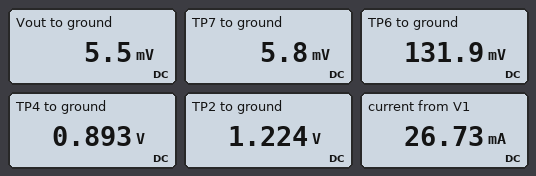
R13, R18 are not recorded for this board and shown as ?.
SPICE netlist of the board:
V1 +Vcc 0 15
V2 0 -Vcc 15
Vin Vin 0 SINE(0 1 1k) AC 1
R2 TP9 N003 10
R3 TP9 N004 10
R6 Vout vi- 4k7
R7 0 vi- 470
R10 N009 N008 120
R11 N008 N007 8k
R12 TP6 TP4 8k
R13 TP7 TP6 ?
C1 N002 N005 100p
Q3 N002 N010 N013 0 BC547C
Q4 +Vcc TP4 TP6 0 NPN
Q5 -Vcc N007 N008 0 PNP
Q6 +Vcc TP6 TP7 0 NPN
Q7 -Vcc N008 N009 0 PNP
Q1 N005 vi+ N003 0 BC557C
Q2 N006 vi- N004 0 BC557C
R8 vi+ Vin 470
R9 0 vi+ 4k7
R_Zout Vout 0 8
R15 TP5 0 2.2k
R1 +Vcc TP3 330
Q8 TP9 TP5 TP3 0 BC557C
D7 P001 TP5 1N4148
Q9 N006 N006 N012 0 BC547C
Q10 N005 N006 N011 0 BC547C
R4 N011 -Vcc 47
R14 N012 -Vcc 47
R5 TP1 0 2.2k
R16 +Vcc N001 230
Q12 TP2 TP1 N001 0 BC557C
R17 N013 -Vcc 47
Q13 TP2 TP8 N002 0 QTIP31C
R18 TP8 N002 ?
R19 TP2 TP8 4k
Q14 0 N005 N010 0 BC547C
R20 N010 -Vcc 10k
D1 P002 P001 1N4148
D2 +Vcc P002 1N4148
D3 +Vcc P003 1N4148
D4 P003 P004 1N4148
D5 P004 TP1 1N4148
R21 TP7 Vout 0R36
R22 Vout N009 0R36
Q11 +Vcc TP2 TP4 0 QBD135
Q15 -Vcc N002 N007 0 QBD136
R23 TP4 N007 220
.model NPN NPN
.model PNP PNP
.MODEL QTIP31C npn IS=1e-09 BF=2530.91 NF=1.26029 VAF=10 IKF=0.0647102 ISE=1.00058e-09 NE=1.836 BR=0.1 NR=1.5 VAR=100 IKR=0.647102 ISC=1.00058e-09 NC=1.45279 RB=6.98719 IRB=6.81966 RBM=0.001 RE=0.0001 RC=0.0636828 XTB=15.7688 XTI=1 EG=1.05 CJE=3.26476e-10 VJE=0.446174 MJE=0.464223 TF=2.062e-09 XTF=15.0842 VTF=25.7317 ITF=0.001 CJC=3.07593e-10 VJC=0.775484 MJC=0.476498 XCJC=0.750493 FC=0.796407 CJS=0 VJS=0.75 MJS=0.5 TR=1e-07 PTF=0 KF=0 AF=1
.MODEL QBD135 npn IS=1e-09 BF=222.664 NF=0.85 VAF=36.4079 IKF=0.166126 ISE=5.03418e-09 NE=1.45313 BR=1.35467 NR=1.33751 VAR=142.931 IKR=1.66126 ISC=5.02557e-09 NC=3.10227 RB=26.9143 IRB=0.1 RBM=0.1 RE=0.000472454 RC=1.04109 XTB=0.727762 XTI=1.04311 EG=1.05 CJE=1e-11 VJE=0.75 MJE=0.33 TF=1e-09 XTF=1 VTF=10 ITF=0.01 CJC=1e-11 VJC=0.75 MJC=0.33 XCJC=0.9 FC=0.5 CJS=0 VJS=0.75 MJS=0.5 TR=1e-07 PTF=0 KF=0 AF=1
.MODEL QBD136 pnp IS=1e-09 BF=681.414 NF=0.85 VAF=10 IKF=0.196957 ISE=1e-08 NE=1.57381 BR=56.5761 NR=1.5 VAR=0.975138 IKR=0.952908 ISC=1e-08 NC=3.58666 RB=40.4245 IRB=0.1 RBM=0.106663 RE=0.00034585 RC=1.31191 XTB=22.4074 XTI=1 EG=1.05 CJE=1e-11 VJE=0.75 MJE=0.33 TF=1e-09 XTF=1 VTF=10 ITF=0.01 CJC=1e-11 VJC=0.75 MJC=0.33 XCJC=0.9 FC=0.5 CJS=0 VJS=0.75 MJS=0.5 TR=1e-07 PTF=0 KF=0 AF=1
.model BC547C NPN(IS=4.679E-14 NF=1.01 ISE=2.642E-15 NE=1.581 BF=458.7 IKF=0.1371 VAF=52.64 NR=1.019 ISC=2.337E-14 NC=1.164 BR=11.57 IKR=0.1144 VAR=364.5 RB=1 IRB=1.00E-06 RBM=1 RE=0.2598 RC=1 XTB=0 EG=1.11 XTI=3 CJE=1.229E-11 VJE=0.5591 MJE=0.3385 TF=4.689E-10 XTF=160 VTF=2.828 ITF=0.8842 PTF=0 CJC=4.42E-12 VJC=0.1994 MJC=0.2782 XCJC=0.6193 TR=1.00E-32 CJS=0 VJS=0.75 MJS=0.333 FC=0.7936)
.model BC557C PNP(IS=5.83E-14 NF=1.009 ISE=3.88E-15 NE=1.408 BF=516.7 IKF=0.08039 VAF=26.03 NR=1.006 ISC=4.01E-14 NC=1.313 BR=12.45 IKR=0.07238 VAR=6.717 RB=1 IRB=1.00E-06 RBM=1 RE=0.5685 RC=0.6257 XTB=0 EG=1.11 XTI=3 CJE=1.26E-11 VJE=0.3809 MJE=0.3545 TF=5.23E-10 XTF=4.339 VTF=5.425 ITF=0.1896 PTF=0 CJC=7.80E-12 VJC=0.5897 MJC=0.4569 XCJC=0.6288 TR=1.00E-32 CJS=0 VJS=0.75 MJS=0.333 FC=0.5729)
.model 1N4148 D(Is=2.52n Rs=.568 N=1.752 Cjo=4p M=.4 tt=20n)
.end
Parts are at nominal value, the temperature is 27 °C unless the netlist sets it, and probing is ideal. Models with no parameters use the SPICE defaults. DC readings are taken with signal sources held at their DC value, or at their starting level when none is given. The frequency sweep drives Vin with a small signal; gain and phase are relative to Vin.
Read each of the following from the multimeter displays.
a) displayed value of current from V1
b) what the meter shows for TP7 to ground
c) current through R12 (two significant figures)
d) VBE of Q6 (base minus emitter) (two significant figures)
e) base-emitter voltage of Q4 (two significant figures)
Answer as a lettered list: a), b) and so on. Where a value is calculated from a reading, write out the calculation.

a) 26.73 mA
b) 5.8 mV
c) (893 mV - 131.9 mV) / 8 kΩ = 95 µA
d) 131.9 mV - 5.8 mV = 130 mV
e) 893 mV - 131.9 mV = 760 mV
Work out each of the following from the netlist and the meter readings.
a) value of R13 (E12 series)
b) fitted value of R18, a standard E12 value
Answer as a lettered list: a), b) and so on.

a) 180 Ω
b) 2.2 kΩ
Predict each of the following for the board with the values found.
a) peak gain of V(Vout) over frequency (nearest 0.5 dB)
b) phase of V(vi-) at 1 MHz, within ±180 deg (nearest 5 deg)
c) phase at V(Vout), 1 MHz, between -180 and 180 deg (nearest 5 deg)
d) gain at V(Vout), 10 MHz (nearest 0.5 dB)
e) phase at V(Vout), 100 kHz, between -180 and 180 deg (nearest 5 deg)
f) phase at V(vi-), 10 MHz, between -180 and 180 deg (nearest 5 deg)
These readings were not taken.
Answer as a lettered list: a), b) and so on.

a) 20.0 dB
b) -85 deg
c) -90 deg
d) -17.0 dB
e) -25 deg
f) 35 deg
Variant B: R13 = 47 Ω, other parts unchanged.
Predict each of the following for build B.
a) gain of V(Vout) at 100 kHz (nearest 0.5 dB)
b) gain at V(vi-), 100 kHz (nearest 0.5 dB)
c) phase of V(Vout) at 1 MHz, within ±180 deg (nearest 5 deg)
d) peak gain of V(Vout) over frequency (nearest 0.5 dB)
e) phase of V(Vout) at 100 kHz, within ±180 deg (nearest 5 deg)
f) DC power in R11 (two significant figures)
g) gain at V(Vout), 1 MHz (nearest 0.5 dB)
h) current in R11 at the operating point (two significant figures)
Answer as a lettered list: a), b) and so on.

a) 20.0 dB
b) -1.0 dB
c) -75 deg
d) 20.0 dB
e) -10 deg
f) 2.9 µW
g) 13.5 dB
h) 19 µA
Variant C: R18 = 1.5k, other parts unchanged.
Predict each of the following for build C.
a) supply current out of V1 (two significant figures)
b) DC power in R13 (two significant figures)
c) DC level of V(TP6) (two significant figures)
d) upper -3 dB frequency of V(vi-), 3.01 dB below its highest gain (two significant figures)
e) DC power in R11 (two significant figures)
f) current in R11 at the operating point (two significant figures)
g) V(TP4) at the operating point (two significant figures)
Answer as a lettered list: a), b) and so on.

a) 29 mA
b) 100 µW
c) 140 mV
d) 220 kHz
e) 24 µW
f) 55 µA
g) 900 mV
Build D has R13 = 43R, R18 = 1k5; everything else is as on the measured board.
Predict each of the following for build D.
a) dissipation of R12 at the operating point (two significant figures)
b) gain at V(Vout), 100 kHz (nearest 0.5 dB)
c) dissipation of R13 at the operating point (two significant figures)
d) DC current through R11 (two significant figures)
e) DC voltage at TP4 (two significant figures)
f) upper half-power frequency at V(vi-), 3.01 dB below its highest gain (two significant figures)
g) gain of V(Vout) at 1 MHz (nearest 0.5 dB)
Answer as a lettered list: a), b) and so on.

a) 73 µW
b) 20.0 dB
c) 25 µW
d) 68 µA
e) 800 mV
f) 550 kHz
g) 14.0 dB
